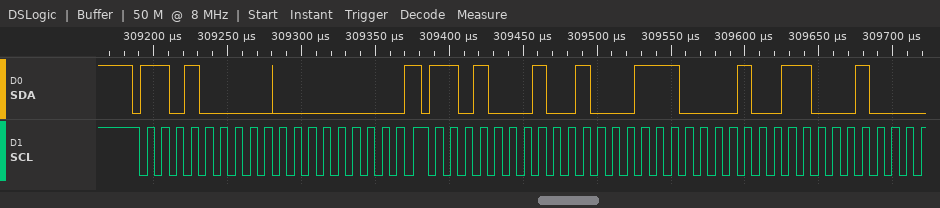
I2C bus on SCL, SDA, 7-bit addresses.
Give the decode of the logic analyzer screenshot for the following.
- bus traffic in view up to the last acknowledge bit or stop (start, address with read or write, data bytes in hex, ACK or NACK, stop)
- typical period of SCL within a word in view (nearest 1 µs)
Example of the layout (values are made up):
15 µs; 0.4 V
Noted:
start, address 68 write ACK, 00 ACK, repeated start, address 68 read ACK, 47 ACK, 13 ACK; 10 µs
